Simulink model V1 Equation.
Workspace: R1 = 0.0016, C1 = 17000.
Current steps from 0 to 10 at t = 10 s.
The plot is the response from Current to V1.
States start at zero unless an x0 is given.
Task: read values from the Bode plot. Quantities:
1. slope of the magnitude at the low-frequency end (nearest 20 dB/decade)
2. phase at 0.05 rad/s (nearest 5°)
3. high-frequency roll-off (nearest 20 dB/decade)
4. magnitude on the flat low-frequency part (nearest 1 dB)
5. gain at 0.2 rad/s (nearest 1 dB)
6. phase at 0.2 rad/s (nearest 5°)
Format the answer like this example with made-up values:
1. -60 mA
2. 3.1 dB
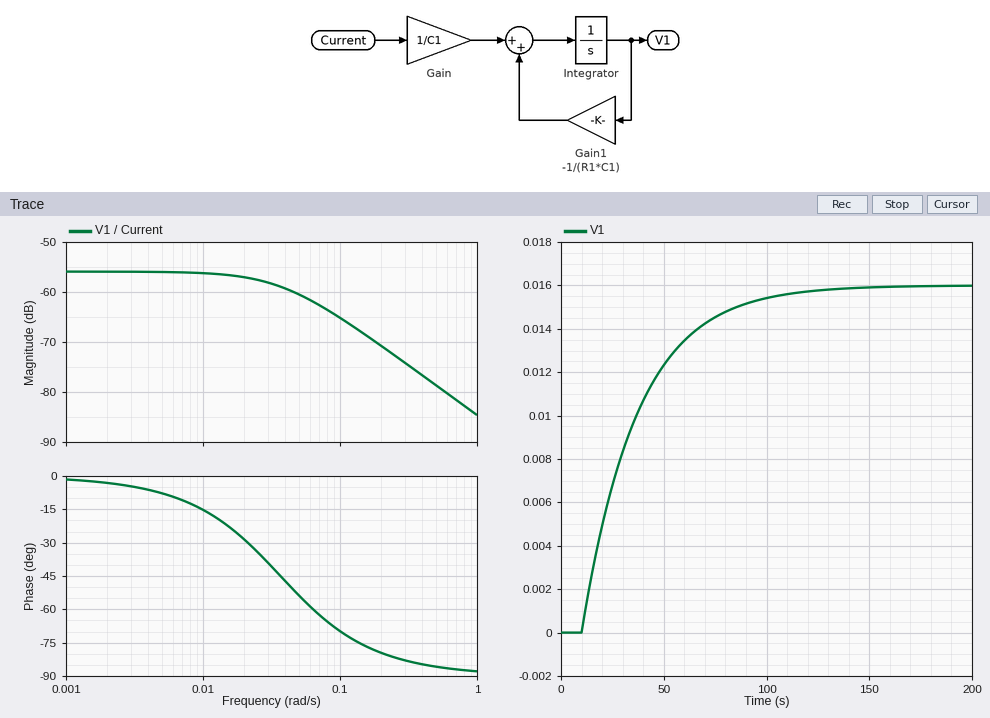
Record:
1. 0 dB/decade
2. -55°
3. -20 dB/decade
4. -56 dB
5. -71 dB
6. -80°
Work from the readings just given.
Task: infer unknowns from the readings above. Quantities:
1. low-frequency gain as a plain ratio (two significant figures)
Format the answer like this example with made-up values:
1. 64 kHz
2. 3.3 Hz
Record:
1. 0.0016
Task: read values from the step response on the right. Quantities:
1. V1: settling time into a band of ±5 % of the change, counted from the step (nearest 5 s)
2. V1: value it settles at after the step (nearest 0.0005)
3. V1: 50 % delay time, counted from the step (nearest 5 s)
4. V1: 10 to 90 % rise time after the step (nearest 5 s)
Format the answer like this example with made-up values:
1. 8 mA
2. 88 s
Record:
1. 80 s
2. 0.0160
3. 20 s
4. 60 s
